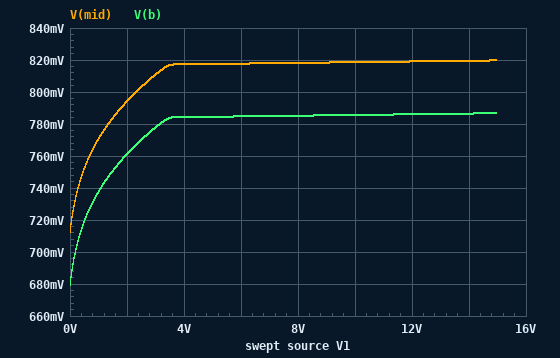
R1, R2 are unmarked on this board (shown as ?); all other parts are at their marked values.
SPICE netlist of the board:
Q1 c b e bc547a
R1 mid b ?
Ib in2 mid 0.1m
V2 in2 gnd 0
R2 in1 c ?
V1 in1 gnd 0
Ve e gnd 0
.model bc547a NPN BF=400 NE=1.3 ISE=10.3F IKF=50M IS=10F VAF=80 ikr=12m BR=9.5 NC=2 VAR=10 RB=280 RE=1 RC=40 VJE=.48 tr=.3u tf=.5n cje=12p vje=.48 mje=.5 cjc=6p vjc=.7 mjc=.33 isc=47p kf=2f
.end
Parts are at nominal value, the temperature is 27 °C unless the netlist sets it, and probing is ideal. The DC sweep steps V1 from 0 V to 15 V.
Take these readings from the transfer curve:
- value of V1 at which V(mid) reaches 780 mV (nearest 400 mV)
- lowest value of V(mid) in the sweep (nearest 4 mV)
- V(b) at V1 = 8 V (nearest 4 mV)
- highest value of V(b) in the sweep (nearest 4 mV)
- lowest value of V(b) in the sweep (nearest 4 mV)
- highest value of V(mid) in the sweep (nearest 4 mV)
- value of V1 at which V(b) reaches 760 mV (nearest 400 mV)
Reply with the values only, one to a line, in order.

1.2 V
712 mV
784 mV
788 mV
680 mV
820 mV
2.0 V
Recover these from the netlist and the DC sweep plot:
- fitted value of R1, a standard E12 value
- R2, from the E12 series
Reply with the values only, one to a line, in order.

330 Ω
150 Ω
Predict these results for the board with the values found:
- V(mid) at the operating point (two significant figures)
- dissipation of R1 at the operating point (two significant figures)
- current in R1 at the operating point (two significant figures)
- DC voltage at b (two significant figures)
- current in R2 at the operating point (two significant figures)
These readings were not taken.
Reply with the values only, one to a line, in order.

710 mV
3.3 µW
100 µA
680 mV
16 µA
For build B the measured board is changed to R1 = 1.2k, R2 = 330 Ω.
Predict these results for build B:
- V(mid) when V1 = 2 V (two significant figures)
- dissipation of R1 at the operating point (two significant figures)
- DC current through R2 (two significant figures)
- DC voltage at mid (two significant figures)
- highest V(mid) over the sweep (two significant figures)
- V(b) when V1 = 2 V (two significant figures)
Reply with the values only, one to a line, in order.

860 mV
12 µW
8.7 µA
800 mV
910 mV
740 mV
